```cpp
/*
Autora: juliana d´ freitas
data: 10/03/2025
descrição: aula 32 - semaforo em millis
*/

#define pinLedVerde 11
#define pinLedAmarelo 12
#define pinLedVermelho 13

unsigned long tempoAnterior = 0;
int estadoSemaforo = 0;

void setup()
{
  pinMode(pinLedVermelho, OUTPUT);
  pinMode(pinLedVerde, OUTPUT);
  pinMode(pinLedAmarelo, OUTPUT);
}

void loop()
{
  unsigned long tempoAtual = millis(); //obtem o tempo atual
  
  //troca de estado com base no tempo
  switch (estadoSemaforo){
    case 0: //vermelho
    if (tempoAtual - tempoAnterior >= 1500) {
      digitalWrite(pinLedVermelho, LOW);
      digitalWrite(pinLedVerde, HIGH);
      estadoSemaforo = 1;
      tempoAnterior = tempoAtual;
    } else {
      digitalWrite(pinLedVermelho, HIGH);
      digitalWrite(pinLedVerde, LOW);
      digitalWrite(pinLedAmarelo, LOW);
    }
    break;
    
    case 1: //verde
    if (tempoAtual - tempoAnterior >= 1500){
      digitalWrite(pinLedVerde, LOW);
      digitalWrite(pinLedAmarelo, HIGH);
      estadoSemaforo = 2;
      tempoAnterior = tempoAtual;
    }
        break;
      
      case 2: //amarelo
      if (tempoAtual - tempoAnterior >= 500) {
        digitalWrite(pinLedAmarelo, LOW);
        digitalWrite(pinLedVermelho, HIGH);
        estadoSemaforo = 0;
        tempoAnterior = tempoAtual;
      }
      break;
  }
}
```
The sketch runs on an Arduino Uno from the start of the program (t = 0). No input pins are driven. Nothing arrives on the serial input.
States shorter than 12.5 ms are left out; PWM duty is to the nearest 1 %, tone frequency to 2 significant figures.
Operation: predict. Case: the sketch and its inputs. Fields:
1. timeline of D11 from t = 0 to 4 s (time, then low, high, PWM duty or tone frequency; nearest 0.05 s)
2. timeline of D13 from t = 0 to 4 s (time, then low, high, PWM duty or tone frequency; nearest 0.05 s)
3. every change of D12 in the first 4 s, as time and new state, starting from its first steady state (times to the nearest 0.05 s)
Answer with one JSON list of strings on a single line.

["0 s low; 1.5 s high; 3 s low", "0 s high; 1.5 s low; 3.5 s high", "0 s low; 3 s high; 3.5 s low"]
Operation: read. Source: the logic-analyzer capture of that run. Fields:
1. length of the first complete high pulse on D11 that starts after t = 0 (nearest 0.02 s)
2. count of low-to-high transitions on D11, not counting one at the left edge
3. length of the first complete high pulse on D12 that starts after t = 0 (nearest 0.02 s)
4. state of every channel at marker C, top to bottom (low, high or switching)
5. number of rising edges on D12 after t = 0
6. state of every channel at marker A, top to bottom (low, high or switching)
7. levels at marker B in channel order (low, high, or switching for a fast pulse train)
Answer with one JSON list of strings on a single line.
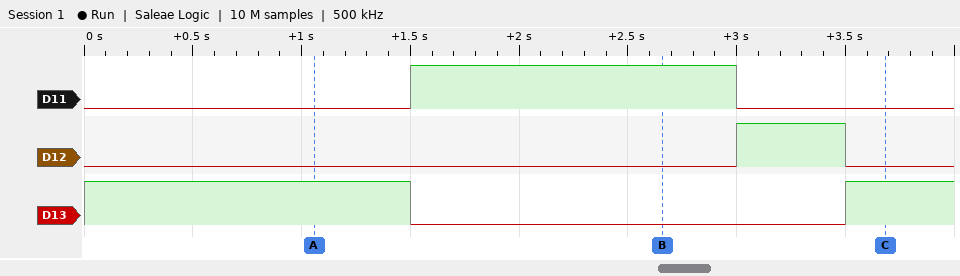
["1.50 s", "1", "0.50 s", "D11 low, D12 low, D13 high", "1", "D11 low, D12 low, D13 high", "D11 high, D12 low, D13 low"]
